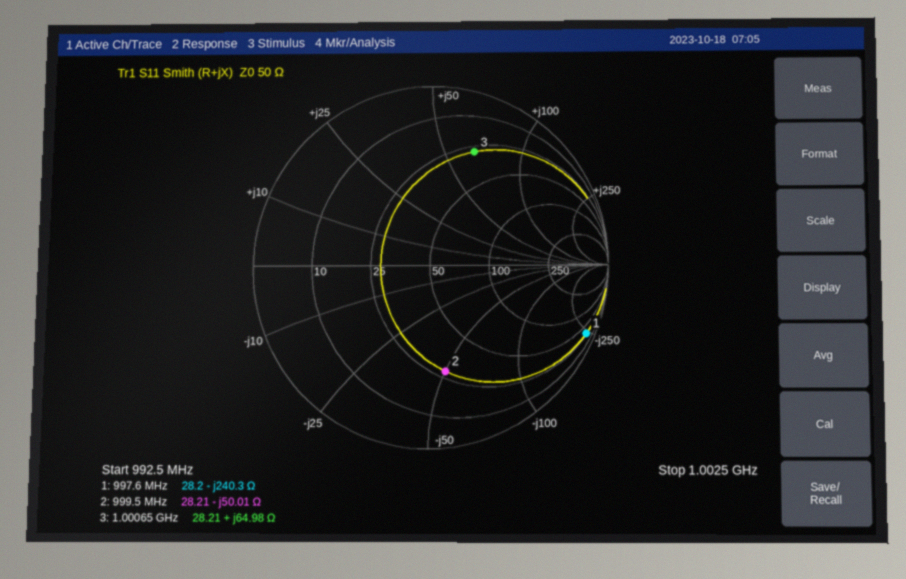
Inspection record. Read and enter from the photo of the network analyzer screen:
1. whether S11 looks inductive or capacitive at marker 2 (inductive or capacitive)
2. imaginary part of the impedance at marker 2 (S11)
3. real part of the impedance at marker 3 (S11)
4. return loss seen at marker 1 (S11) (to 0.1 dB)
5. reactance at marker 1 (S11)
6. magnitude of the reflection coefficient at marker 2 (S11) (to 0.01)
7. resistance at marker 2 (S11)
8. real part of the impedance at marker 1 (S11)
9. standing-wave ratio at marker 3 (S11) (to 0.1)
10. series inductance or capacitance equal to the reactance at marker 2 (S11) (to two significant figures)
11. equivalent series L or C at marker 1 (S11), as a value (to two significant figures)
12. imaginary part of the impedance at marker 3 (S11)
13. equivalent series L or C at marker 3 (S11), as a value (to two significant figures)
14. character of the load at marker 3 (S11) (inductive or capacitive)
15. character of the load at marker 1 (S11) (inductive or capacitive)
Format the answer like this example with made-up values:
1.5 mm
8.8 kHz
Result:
capacitive
-50.01 Ω
28.21 Ω
0.4 dB
-240.3 Ω
0.59
28.21 Ω
28.2 Ω
5.1
3.2 pF
660 fF
+64.98 Ω
10 nH
inductive
capacitive
